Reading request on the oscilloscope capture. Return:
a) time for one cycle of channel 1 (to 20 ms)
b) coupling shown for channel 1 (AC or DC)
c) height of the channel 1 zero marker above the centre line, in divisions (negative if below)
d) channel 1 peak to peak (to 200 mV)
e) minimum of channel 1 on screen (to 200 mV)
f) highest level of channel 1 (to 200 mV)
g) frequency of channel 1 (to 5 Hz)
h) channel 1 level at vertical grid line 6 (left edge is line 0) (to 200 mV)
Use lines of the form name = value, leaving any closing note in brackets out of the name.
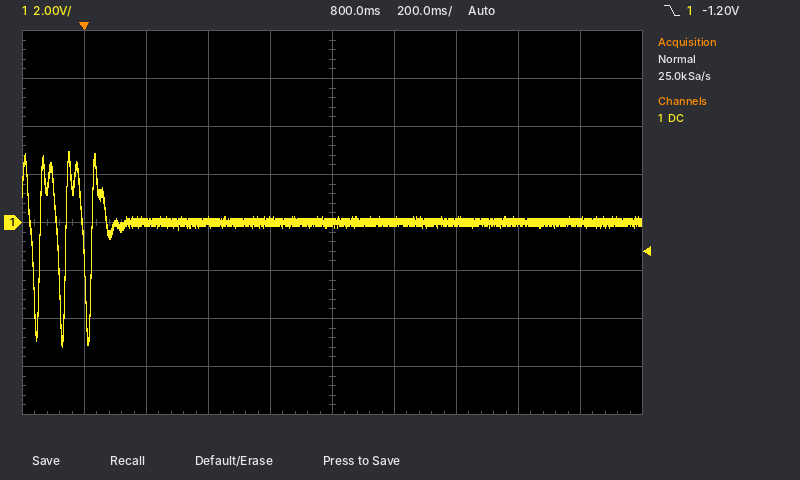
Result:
time for one cycle of channel 1 = 80 ms
coupling shown for channel 1 = DC
height of the channel 1 zero marker above the centre line, in divisions = 0.0 div
channel 1 peak to peak = 8.2 V
minimum of channel 1 on screen = -5.2 V
highest level of channel 1 = 3.0 V
frequency of channel 1 = 10 Hz
channel 1 level at vertical grid line 6 (left edge is line 0) = 0.0 V
